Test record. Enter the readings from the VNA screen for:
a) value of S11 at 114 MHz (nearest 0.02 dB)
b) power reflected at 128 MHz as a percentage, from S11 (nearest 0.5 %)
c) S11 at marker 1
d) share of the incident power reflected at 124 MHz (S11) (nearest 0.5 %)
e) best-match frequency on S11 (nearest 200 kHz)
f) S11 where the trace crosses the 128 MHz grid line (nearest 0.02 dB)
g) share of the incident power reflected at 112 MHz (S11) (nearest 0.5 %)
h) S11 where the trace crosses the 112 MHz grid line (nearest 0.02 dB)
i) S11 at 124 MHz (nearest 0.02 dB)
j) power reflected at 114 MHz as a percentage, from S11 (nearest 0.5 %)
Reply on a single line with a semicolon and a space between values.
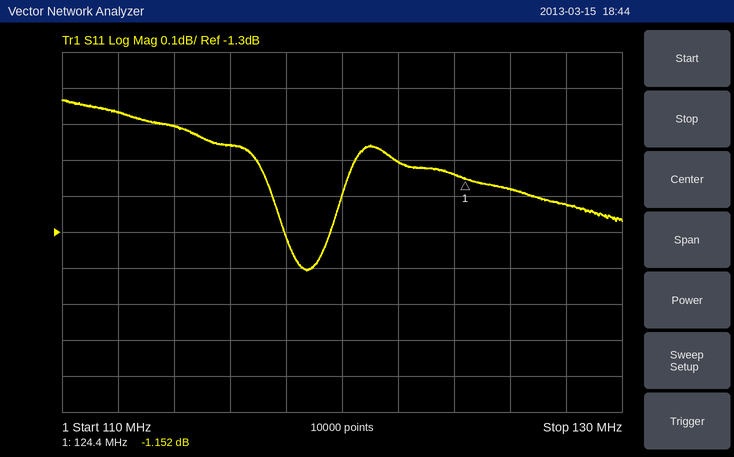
-1.00 dB; 75.5 %; -1.152 dB; 77.0 %; 118.8 MHz; -1.22 dB; 80.0 %; -0.96 dB; -1.14 dB; 79.5 %
